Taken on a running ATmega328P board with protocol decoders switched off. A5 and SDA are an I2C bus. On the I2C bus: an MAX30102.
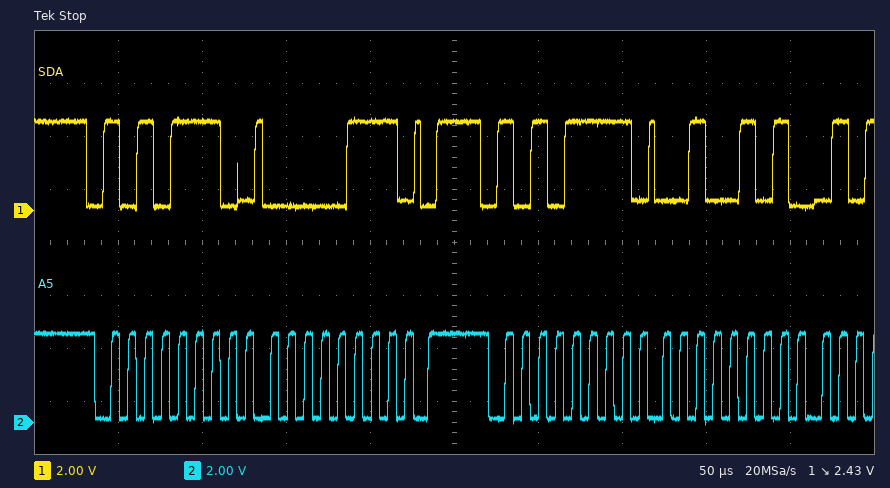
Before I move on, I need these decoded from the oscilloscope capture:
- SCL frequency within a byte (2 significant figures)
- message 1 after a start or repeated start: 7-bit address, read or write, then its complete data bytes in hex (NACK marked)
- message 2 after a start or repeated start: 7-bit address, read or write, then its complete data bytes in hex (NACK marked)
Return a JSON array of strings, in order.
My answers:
["100 kHz", "0x57 write: 07", "0x57 read: 25"]
